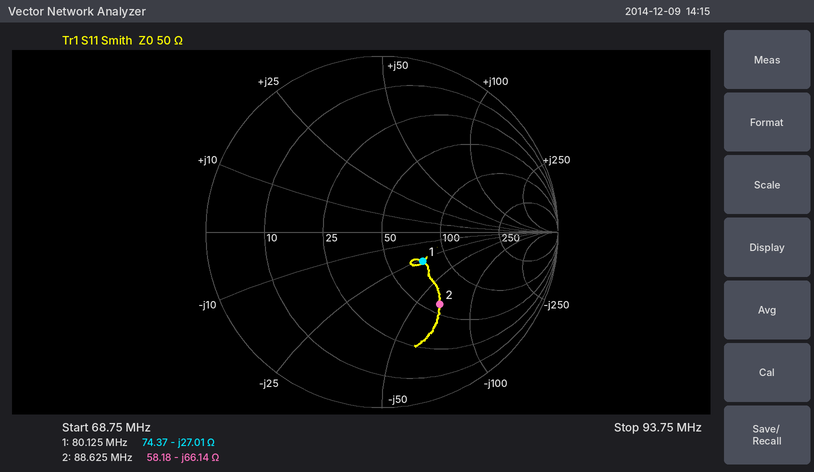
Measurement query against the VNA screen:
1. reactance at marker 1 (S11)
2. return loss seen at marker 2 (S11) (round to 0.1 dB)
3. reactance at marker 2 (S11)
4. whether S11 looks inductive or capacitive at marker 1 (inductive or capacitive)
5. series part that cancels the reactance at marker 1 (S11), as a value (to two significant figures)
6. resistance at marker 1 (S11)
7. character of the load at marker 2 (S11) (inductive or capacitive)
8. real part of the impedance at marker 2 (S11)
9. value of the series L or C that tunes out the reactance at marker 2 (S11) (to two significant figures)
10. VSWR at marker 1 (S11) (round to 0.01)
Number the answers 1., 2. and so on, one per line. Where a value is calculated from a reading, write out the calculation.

1. -27.01 Ω
2. 5.6 dB
3. -66.14 Ω
4. capacitive
5. L = 27.01 Ω/(2π × 80.125 MHz) ≈ 54 nH
6. 74.37 Ω
7. capacitive
8. 58.18 Ω
9. L = 66.14 Ω/(2π × 88.625 MHz) ≈ 119 nH, so 120 nH to two significant figures
10. 1.80
